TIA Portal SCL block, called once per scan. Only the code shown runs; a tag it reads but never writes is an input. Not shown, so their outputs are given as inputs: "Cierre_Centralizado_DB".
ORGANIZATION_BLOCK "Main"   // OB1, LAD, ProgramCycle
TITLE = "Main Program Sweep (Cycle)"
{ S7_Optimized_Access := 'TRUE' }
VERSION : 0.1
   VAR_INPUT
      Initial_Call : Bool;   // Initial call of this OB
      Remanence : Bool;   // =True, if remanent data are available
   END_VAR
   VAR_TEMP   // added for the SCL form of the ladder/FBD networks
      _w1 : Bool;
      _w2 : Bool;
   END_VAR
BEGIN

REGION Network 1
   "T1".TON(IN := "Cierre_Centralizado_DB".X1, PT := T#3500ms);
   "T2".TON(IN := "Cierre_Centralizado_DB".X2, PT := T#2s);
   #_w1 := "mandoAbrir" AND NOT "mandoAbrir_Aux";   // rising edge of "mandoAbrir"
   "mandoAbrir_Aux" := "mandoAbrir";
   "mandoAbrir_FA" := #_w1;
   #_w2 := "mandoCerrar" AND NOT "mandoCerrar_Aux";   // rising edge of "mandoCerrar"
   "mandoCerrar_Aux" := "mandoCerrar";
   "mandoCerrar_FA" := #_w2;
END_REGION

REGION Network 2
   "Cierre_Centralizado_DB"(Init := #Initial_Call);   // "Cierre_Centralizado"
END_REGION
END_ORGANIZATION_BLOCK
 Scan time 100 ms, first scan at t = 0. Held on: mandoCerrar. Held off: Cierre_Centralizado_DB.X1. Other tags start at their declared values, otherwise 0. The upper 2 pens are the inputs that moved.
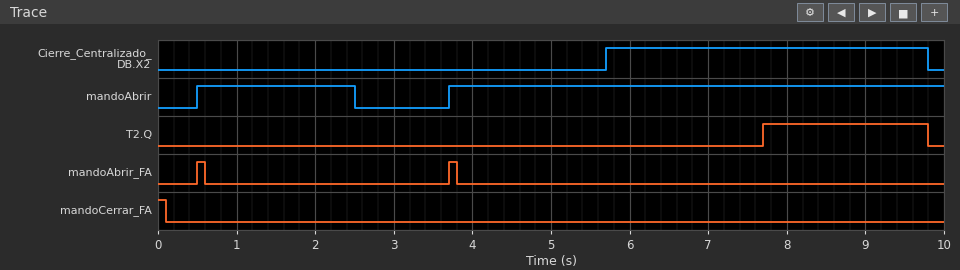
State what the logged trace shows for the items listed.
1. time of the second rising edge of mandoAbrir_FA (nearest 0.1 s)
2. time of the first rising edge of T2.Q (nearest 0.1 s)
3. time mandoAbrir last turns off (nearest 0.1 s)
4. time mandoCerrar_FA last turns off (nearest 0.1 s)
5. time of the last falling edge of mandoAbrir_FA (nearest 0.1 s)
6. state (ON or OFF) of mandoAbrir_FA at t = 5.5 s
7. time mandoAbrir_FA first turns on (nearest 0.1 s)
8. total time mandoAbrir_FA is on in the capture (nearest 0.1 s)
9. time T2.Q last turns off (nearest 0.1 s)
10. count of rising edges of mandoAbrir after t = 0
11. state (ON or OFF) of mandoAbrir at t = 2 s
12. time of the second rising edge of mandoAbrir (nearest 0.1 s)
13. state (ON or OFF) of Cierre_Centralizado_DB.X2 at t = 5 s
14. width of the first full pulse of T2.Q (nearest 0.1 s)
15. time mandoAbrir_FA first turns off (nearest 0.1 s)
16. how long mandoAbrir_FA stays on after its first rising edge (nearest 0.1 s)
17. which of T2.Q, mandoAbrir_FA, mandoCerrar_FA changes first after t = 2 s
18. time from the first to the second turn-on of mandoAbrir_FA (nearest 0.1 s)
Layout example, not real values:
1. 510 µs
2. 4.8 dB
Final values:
1. 3.7 s
2. 7.7 s
3. 2.5 s
4. 0.1 s
5. 3.8 s
6. OFF
7. 0.5 s
8. 0.2 s
9. 9.8 s
10. 2
11. ON
12. 3.7 s
13. OFF
14. 2.1 s
15. 0.6 s
16. 0.1 s
17. mandoAbrir_FA
18. 3.2 s
